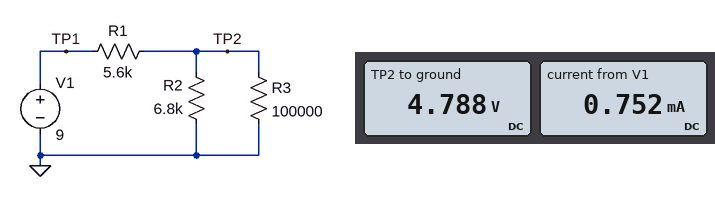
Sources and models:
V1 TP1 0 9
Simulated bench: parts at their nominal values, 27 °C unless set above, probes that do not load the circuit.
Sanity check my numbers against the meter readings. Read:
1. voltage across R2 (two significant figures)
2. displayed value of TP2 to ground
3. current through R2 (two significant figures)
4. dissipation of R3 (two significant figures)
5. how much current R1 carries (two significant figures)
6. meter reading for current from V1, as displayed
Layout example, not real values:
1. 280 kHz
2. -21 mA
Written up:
1. 4.8 V
2. 4.788 V
3. 700 µA
4. 230 µW
5. 750 µA
6. 0.752 mA
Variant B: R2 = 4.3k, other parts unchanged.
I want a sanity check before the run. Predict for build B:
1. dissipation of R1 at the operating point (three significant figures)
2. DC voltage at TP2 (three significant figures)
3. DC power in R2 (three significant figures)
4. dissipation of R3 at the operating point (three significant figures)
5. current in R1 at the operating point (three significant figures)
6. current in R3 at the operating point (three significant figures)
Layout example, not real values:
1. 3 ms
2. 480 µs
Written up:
1. 4.80 mW
2. 3.82 V
3. 3.39 mW
4. 146 µW
5. 926 µA
6. 38.2 µA
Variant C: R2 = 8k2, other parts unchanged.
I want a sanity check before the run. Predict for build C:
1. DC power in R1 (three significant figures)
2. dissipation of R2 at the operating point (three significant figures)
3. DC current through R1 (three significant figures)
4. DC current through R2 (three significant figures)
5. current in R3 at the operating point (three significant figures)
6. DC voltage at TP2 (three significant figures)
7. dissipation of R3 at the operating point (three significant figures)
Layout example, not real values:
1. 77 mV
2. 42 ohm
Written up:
1. 2.61 mW
2. 3.27 mW
3. 683 µA
4. 631 µA
5. 51.8 µA
6. 5.18 V
7. 268 µW
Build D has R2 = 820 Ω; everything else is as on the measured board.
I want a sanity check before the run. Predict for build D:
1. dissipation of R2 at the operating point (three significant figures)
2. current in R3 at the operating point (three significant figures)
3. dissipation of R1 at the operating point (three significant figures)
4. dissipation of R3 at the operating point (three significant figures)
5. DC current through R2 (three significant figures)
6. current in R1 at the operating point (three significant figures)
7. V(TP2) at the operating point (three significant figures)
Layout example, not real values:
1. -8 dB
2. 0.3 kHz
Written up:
1. 1.59 mW
2. 11.4 µA
3. 11.0 mW
4. 13.0 µW
5. 1.39 mA
6. 1.40 mA
7. 1.14 V
